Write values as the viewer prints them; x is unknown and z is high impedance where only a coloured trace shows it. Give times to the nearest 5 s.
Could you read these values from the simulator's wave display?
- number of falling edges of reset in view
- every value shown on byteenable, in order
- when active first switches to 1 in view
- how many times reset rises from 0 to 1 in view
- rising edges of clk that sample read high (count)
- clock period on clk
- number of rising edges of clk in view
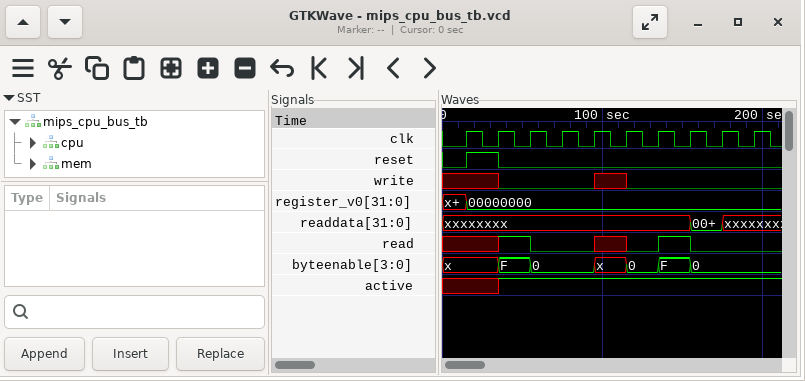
1
x, F, 0, x, 0, F, 0
35 s
1
2
20 s
10
